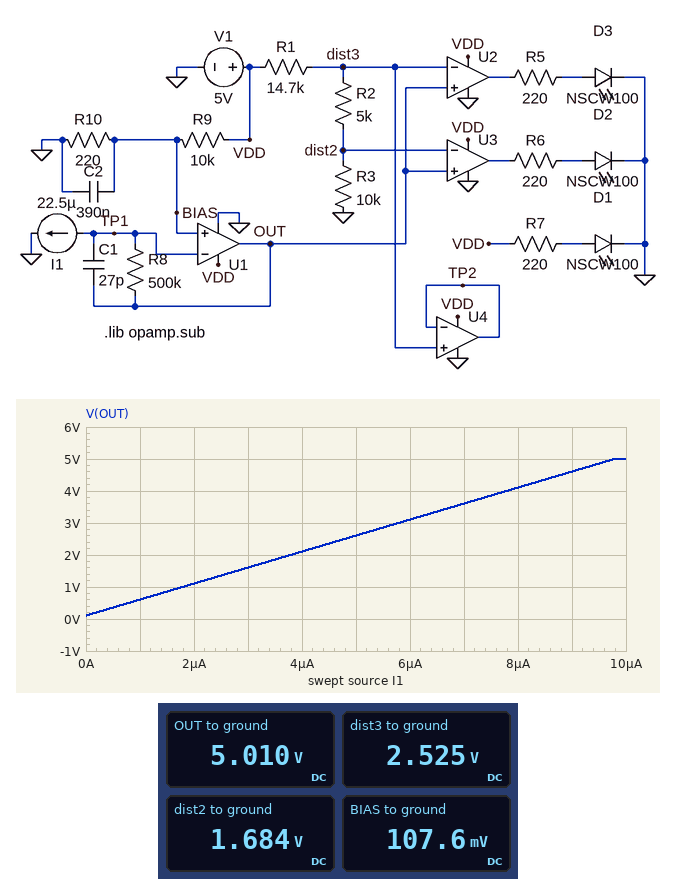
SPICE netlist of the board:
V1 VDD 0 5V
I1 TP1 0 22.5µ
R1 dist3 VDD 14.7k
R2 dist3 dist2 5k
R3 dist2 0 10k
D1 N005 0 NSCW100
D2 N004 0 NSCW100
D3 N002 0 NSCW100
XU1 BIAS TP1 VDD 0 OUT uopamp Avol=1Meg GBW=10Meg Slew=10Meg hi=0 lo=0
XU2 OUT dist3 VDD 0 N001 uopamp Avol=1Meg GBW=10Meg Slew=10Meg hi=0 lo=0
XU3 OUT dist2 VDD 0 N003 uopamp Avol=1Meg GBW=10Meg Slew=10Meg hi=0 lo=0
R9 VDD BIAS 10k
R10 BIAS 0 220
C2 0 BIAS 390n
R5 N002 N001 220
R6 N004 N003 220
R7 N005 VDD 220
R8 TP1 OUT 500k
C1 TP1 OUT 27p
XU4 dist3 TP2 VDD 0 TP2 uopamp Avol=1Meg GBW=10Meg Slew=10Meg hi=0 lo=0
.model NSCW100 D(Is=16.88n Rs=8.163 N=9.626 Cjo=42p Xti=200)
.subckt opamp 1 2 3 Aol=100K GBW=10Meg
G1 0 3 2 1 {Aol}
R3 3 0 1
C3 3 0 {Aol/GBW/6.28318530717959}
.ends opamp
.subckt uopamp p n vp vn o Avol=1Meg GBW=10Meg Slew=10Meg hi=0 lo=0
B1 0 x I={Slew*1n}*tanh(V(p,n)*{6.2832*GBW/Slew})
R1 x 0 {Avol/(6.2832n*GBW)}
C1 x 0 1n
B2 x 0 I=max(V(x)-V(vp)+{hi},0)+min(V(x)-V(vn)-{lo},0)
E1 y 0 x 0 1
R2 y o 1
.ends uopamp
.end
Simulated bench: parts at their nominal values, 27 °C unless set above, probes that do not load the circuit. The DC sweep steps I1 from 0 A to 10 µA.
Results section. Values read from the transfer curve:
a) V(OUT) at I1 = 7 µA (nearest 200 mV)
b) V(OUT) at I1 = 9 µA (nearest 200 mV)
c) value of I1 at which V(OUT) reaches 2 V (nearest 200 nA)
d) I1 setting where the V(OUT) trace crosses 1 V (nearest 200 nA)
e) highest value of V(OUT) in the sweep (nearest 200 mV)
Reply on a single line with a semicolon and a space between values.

3.6 V; 4.6 V; 3.8 µA; 1.8 µA; 5.0 V
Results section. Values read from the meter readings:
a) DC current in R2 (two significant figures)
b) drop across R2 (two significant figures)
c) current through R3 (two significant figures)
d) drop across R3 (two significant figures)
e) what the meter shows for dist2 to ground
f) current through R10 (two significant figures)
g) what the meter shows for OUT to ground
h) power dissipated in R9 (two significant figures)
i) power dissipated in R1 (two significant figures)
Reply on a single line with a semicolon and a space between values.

170 µA; 840 mV; 170 µA; 1.7 V; 1.684 V; 490 µA; 5.010 V; 2.4 mW; 420 µW
